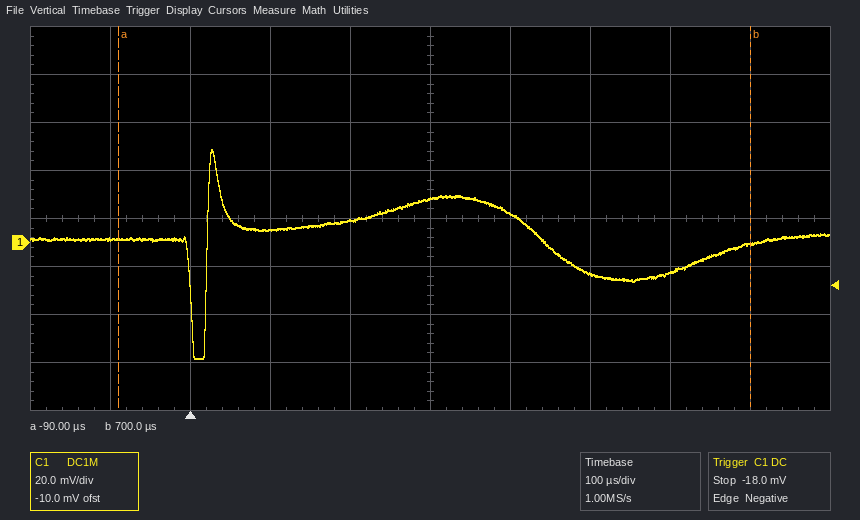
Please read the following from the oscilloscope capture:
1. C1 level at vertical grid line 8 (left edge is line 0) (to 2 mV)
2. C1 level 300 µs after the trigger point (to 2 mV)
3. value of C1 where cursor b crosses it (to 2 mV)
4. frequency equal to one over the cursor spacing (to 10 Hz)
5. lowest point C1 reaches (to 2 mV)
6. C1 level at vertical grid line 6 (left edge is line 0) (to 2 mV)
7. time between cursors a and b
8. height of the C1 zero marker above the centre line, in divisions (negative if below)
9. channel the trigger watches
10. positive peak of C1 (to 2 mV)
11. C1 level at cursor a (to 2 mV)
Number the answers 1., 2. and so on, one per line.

1. -12 mV
2. 18 mV
3. 0 mV
4. 1.27 kHz
5. -48 mV
6. 12 mV
7. 790 µs
8. -0.5 div
9. C1
10. 38 mV
11. 2 mV
